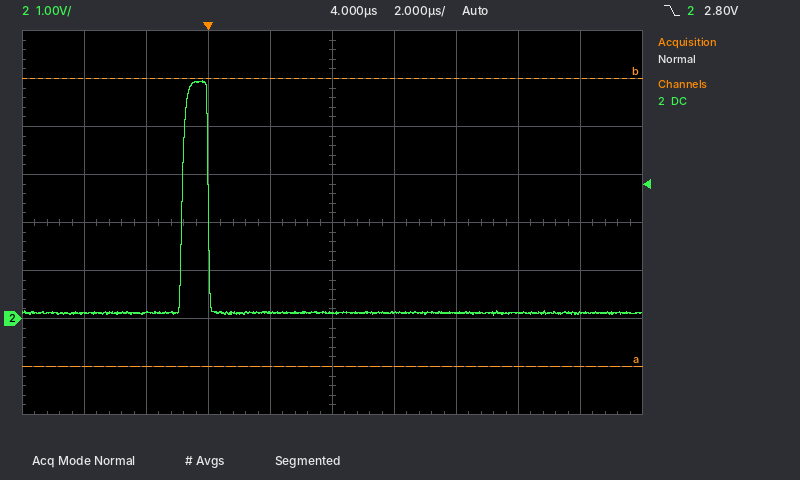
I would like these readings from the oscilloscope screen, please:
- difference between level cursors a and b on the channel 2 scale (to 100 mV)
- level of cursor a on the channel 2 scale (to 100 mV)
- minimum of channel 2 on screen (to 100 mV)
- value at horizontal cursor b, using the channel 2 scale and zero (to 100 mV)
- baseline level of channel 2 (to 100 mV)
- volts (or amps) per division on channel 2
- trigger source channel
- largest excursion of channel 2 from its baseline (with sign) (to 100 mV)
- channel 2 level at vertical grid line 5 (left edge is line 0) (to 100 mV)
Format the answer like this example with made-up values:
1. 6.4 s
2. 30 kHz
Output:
1. 6.0 V
2. -1.0 V
3. 100 mV
4. 5.0 V
5. 100 mV
6. 1 V
7. channel 2
8. +4.8 V
9. 100 mV
